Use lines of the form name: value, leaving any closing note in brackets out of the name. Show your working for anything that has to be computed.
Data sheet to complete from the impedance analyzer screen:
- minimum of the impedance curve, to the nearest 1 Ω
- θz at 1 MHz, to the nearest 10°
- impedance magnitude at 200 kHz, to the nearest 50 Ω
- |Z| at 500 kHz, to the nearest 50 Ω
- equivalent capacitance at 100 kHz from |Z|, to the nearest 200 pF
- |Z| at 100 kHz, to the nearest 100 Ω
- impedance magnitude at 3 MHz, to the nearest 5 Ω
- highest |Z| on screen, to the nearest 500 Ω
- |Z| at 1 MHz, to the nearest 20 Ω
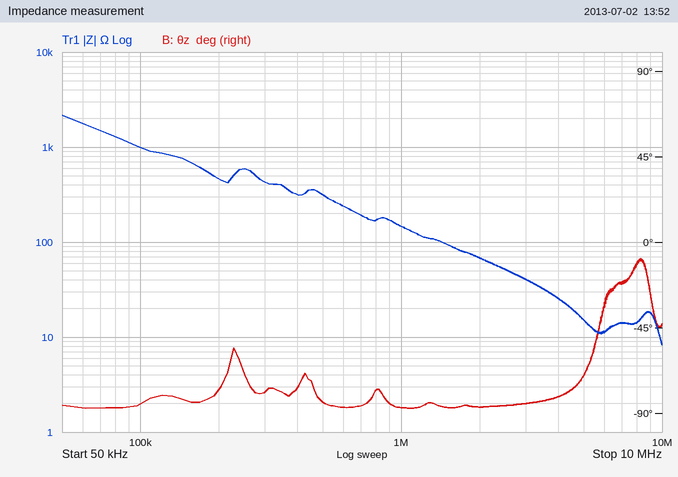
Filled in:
minimum of the impedance curve, to the nearest 1 Ω: 8 Ω
θz at 1 MHz, to the nearest 10°: -90°
impedance magnitude at 200 kHz, to the nearest 50 Ω: 450 Ω
|Z| at 500 kHz, to the nearest 50 Ω: 300 Ω
equivalent capacitance at 100 kHz from |Z|, to the nearest 200 pF: C = 1/(2π × 100 kHz × 1.0 kΩ) ≈ 1.6 nF
|Z| at 100 kHz, to the nearest 100 Ω: 1.0 kΩ
impedance magnitude at 3 MHz, to the nearest 5 Ω: 40 Ω
highest |Z| on screen, to the nearest 500 Ω: 2.0 kΩ
|Z| at 1 MHz, to the nearest 20 Ω: 140 Ω
